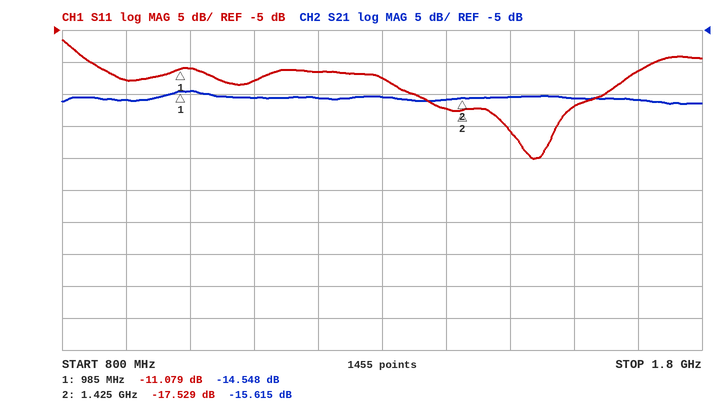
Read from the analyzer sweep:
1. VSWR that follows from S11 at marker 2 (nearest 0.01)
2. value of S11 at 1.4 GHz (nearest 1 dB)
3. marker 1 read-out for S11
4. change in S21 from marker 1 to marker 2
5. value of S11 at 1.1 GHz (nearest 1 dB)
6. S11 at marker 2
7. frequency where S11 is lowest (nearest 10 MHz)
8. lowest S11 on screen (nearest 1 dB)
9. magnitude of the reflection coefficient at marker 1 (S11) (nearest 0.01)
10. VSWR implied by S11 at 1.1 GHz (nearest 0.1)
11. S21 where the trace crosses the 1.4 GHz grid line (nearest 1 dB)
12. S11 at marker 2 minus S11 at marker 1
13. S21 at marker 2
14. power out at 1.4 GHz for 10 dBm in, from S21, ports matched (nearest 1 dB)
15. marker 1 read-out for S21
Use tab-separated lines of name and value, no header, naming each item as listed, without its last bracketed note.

VSWR that follows from S11 at marker 2	1.31
value of S11 at 1.4 GHz	-17 dB
marker 1 read-out for S11	-11.079 dB
change in S21 from marker 1 to marker 2	-1.067 dB
value of S11 at 1.1 GHz	-13 dB
S11 at marker 2	-17.529 dB
frequency where S11 is lowest	1.54 GHz
lowest S11 on screen	-25 dB
magnitude of the reflection coefficient at marker 1 (S11)	0.28
VSWR implied by S11 at 1.1 GHz	1.6
S21 where the trace crosses the 1.4 GHz grid line	-16 dB
S11 at marker 2 minus S11 at marker 1	-6.450 dB
S21 at marker 2	-15.615 dB
power out at 1.4 GHz for 10 dBm in, from S21, ports matched	-6 dBm
marker 1 read-out for S21	-14.548 dB
